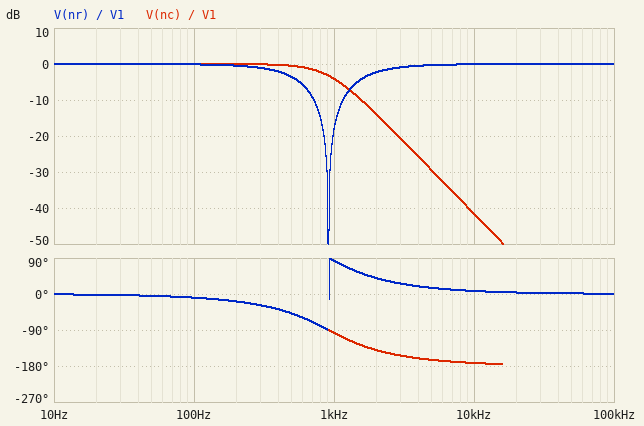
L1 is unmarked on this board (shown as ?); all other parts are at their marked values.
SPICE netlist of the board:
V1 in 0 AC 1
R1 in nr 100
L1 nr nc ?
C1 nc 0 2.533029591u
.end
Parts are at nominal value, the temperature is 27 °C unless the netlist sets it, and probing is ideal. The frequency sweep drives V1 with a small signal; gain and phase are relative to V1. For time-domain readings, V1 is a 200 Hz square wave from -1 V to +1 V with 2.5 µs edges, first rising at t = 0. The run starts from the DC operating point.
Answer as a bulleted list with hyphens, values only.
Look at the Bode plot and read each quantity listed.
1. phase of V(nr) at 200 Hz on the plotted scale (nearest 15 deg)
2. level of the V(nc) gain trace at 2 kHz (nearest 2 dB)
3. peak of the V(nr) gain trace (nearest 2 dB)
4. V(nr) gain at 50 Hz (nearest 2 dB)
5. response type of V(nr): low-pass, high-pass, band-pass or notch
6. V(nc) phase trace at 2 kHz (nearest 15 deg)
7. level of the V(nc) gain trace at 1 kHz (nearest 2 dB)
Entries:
- -15 deg
- -14 dB
- 0 dB
- 0 dB
- notch
- -135 deg
- -4 dB
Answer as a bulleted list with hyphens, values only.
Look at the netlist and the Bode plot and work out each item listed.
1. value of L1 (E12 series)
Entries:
- 12 mH
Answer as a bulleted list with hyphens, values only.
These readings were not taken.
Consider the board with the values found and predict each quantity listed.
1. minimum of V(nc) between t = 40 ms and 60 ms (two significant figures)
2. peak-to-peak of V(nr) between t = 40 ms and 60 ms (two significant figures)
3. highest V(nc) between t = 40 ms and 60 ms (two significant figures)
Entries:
- -1.1 V
- 2.1 V
- 1.1 V
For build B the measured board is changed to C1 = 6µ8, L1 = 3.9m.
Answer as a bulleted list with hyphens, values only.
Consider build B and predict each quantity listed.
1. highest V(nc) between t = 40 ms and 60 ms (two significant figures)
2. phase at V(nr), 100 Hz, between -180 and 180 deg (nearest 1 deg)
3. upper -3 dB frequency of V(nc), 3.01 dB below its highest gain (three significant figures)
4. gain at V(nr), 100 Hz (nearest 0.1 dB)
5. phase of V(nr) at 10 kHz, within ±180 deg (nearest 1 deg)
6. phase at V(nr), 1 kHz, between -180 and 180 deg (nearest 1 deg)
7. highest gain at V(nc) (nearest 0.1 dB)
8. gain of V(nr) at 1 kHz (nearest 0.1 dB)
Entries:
- 960 mV
- -23 deg
- 248 Hz
- -0.7 dB
- 22 deg
- 89 deg
- 0 dB
- -39.2 dB
